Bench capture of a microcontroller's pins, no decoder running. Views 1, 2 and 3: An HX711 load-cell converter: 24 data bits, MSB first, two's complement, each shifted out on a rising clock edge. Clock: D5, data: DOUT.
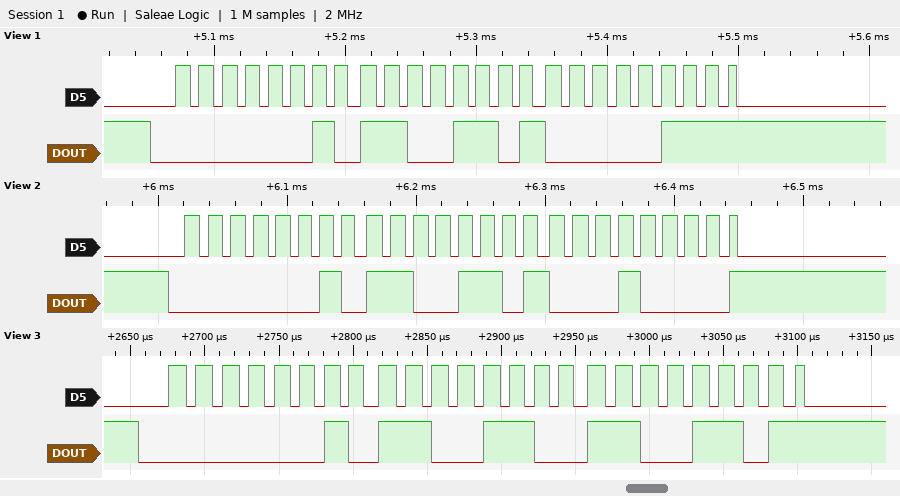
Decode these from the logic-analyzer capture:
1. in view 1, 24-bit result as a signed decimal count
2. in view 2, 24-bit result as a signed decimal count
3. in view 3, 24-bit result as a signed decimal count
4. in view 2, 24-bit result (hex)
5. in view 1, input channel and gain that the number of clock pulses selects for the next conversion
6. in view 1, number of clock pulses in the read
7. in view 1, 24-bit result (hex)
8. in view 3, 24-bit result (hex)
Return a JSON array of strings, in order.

["183559", "183568", "183501", "0x02CD10", "channel A, gain 128", "25", "0x02CD07", "0x02CCCD"]
